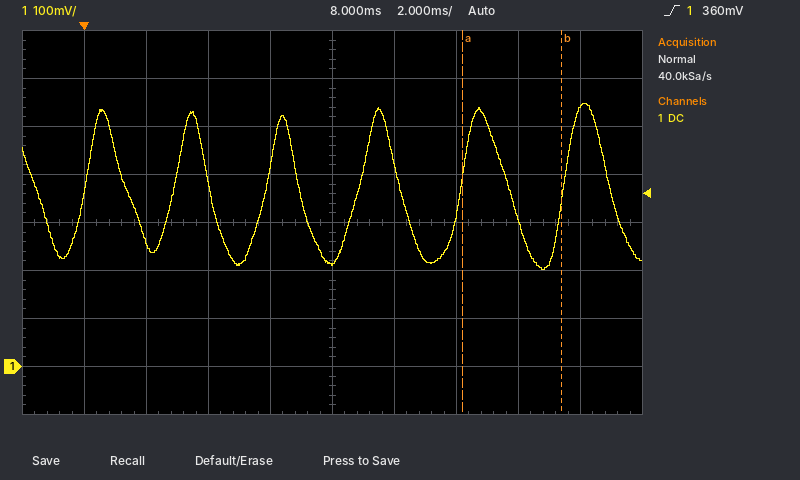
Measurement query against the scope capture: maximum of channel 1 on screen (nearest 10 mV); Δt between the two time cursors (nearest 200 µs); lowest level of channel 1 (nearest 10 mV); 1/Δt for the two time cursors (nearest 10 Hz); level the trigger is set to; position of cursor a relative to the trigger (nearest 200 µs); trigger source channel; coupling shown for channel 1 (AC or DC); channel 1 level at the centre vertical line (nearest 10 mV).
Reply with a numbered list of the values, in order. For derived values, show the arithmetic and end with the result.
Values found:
1. 550 mV
2. 3.2 ms
3. 200 mV
4. 1 / 3.2 ms ≈ 310 Hz
5. 360 mV
6. +12.2 ms
7. channel 1
8. DC
9. 210 mV
